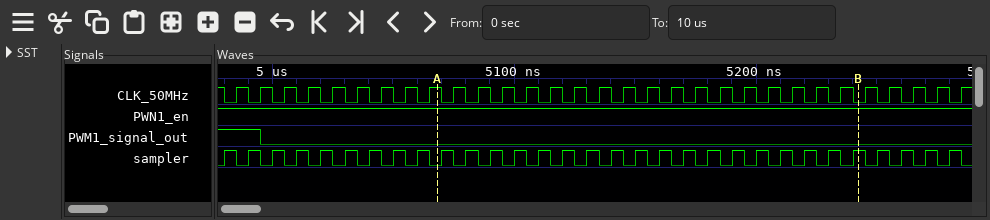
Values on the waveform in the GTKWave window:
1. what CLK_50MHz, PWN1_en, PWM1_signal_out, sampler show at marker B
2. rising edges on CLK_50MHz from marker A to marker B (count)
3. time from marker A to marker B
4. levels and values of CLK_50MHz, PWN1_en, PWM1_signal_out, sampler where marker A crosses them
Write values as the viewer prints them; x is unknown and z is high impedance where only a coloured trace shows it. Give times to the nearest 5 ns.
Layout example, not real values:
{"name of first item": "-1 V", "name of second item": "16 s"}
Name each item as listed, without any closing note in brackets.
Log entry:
{"what CLK_50MHz, PWN1_en, PWM1_signal_out, sampler show at marker B": "CLK_50MHz=0, PWN1_en=1, PWM1_signal_out=0, sampler=1", "rising edges on CLK_50MHz from marker A to marker B": "17", "time from marker A to marker B": "175 ns", "levels and values of CLK_50MHz, PWN1_en, PWM1_signal_out, sampler where marker A crosses them": "CLK_50MHz=1, PWN1_en=1, PWM1_signal_out=0, sampler=0"}
